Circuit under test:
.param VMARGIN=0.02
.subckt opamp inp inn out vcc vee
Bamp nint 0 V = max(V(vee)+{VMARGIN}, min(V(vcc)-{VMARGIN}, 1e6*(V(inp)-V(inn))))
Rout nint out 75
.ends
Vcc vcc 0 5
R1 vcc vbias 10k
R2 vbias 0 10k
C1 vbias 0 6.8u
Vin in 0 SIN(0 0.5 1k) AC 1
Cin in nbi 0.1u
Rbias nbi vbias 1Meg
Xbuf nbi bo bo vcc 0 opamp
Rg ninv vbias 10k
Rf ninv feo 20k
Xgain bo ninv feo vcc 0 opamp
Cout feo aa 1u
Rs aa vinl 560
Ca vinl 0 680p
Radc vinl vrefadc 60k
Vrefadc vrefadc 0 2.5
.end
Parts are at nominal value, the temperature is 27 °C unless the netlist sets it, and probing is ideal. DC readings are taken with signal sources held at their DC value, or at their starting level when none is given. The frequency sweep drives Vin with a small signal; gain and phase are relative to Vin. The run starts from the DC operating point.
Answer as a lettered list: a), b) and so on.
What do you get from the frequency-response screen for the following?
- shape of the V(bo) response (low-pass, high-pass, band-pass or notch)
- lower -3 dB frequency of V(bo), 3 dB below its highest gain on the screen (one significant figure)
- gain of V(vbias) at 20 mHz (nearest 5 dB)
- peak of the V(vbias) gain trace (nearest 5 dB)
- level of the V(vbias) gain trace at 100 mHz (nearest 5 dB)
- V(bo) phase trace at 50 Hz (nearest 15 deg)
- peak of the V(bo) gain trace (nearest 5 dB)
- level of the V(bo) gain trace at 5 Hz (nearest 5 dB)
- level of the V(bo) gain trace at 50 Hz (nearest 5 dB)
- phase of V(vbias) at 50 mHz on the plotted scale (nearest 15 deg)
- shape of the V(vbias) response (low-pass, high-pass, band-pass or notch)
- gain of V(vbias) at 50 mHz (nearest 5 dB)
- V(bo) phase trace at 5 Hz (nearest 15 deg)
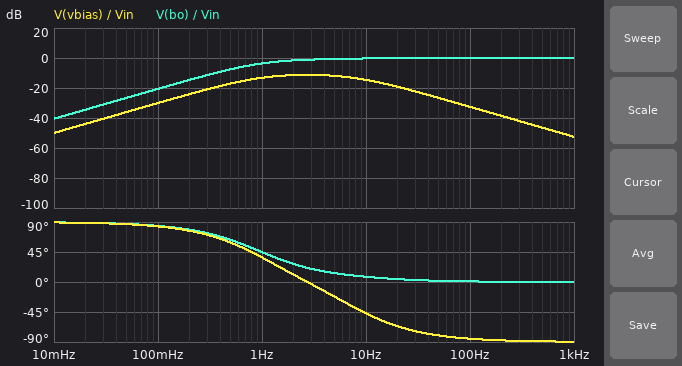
a) high-pass
b) 1 Hz
c) -45 dB
d) -10 dB
e) -30 dB
f) 0 deg
g) 0 dB
h) 0 dB
i) 0 dB
j) 90 deg
k) band-pass
l) -35 dB
m) 15 deg
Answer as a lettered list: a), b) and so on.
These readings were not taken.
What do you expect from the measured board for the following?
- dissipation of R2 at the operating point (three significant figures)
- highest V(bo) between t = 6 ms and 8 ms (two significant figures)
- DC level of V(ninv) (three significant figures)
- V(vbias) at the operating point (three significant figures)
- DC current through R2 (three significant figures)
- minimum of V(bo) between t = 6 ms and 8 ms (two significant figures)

a) 625 µW
b) 3.0 V
c) 2.50 V
d) 2.50 V
e) 250 µA
f) 2.0 V
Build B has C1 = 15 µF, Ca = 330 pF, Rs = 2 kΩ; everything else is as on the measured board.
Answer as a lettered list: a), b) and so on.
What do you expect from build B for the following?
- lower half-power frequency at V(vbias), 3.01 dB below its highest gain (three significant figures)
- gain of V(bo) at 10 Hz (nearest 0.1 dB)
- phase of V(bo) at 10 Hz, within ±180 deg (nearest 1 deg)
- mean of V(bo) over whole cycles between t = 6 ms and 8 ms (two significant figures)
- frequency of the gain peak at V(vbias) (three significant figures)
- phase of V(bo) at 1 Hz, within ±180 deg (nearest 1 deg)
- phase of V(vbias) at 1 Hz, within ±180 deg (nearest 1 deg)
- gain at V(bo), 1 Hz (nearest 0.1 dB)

a) 624 mHz
b) -0.2 dB
c) 9 deg
d) 2.5 V
e) 1.84 Hz
f) 44 deg
g) 26 deg
h) -4.1 dB
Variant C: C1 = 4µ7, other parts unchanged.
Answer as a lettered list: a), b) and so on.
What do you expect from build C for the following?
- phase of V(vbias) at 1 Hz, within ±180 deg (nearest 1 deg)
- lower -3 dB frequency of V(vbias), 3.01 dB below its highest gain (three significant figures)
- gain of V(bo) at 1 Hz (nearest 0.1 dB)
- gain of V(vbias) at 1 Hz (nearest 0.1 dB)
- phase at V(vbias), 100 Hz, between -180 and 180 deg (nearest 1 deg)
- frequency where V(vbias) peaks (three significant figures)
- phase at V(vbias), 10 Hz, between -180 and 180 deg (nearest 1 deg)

a) 40 deg
b) 853 mHz
c) -3.5 dB
d) -13.0 dB
e) -83 deg
f) 3.28 Hz
g) -37 deg
